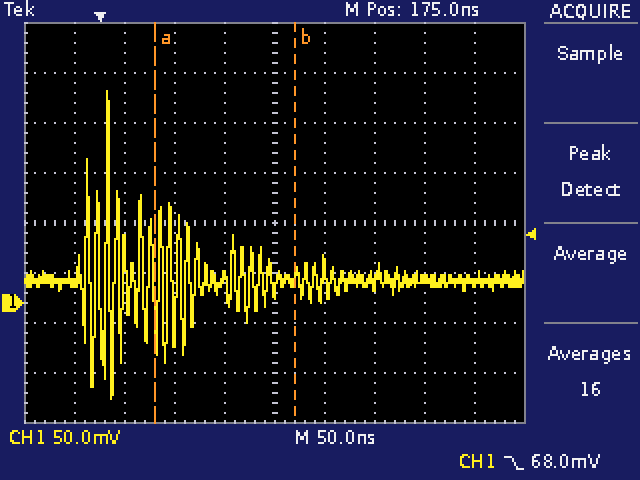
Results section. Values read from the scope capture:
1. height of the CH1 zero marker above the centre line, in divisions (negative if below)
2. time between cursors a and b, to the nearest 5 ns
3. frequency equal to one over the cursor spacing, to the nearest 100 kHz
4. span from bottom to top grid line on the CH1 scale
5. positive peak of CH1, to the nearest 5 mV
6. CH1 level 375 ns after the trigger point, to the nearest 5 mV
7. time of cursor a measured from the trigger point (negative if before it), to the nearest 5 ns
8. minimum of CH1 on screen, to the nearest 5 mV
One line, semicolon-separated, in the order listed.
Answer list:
-1.6 div; 140 ns; 7.1 MHz; 400 mV; 210 mV; 20 mV; +55 ns; -95 mV
